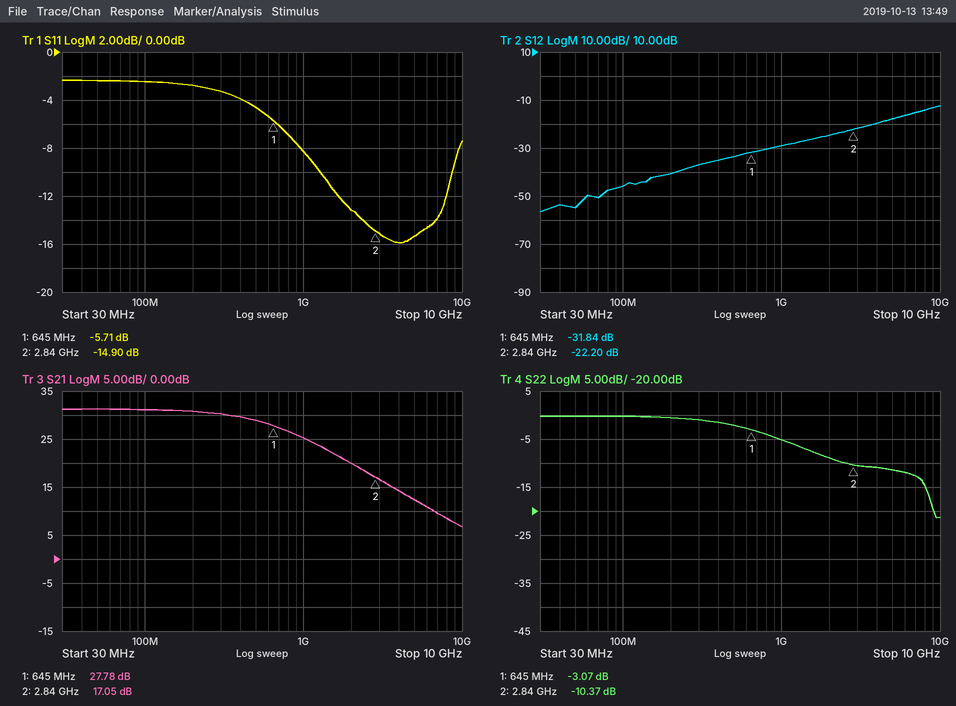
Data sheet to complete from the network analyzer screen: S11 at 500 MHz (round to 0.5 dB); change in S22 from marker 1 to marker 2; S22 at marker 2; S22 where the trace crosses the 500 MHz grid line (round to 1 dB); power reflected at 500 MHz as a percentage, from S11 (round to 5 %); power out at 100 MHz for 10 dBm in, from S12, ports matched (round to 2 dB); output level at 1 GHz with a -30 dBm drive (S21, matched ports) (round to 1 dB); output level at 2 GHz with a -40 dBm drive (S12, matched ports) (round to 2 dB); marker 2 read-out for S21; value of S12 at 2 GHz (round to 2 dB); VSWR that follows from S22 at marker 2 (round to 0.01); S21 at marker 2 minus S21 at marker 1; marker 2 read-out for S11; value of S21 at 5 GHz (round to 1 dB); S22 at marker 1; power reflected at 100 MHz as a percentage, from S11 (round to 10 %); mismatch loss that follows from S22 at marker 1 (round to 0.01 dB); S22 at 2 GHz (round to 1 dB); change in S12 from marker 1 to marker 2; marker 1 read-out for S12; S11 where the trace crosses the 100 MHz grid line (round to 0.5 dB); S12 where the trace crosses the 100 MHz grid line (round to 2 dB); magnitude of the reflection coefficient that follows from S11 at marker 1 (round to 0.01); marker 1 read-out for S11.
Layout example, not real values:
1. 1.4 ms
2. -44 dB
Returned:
1. -4.5 dB
2. -7.30 dB
3. -10.37 dB
4. -2 dB
5. 35 %
6. -36 dBm
7. -5 dBm
8. -64 dBm
9. 17.05 dB
10. -24 dB
11. 1.87
12. -10.73 dB
13. -14.90 dB
14. 12 dB
15. -3.07 dB
16. 60 %
17. 2.95 dB
18. -9 dB
19. 9.64 dB
20. -31.84 dB
21. -2.5 dB
22. -46 dB
23. 0.52
24. -5.71 dB
